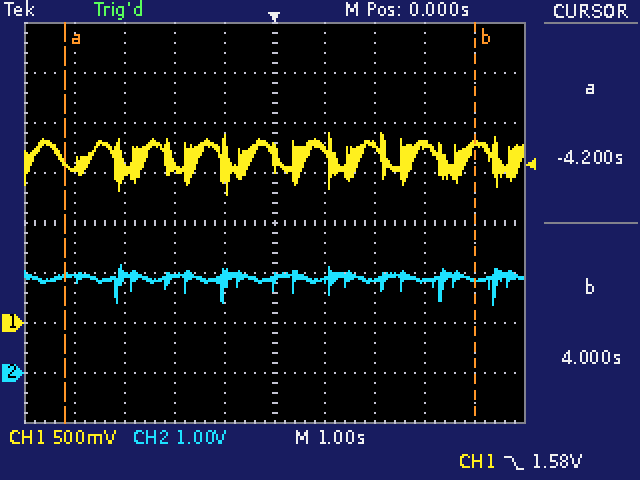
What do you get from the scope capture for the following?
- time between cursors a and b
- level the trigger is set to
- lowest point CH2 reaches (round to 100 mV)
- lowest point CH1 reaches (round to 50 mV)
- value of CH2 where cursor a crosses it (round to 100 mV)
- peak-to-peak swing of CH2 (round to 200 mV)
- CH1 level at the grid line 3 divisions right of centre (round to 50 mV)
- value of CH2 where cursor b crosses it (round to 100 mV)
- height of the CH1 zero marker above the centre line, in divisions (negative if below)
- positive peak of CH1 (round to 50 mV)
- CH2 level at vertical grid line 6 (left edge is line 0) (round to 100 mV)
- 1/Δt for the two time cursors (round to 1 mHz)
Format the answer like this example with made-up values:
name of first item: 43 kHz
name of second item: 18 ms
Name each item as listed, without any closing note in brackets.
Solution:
time between cursors a and b: 8.2 s
level the trigger is set to: 1.58 V
lowest point CH2 reaches: 1.4 V
lowest point CH1 reaches: 1.30 V
value of CH2 where cursor a crosses it: 1.9 V
peak-to-peak swing of CH2: 800 mV
CH1 level at the grid line 3 divisions right of centre: 1.80 V
value of CH2 where cursor b crosses it: 1.9 V
height of the CH1 zero marker above the centre line, in divisions: -2.0 div
positive peak of CH1: 1.90 V
CH2 level at vertical grid line 6 (left edge is line 0): 1.9 V
1/Δt for the two time cursors: 122 mHz
